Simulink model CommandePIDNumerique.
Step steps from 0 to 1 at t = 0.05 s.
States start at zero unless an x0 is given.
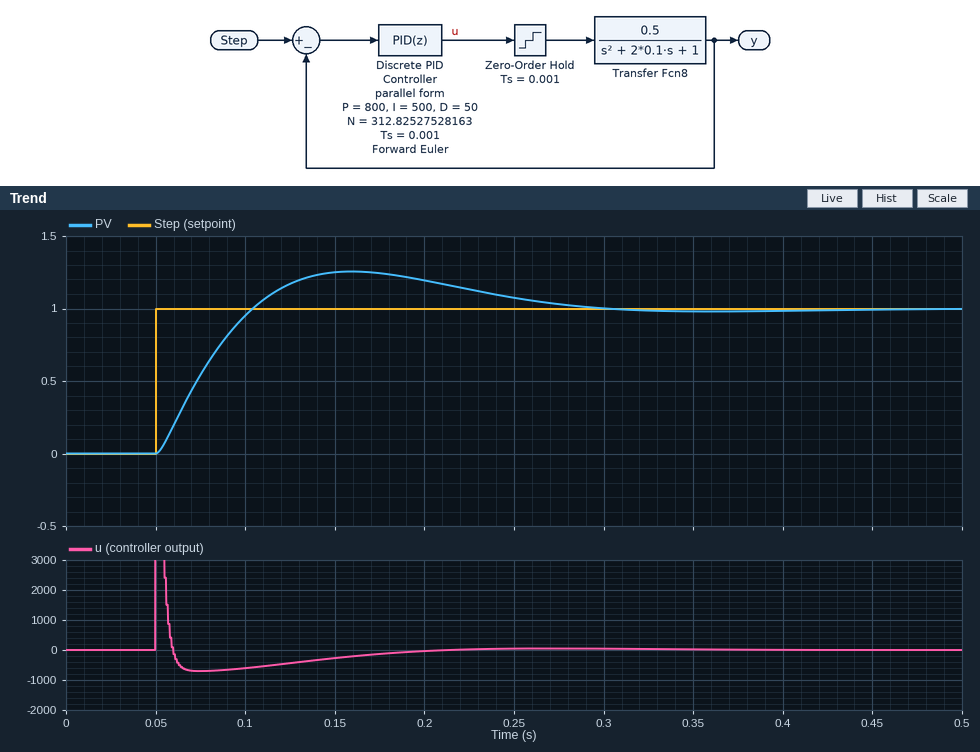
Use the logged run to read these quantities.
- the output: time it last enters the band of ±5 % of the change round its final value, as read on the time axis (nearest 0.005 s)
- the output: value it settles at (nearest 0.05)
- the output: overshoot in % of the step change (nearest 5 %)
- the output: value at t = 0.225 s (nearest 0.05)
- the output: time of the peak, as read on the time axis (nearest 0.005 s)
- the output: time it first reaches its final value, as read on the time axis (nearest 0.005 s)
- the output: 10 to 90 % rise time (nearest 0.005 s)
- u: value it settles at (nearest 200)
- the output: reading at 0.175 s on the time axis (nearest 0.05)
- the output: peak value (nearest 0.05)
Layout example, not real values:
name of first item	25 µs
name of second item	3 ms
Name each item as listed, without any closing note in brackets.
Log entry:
the output: time it last enters the band of ±5 % of the change round its final value, as read on the time axis	0.265 s
the output: value it settles at	1.00
the output: overshoot in % of the step change	25 %
the output: value at t = 0.225 s	1.15
the output: time of the peak, as read on the time axis	0.160 s
the output: time it first reaches its final value, as read on the time axis	0.105 s
the output: 10 to 90 % rise time	0.040 s
u: value it settles at	0
the output: reading at 0.175 s on the time axis	1.25
the output: peak value	1.25
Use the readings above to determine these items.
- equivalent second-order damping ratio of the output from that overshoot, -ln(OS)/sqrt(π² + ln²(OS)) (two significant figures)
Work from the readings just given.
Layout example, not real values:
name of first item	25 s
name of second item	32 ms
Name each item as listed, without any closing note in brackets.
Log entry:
equivalent second-order damping ratio of the output from that overshoot, -ln(OS)/sqrt(π² + ln²(OS))	0.40
